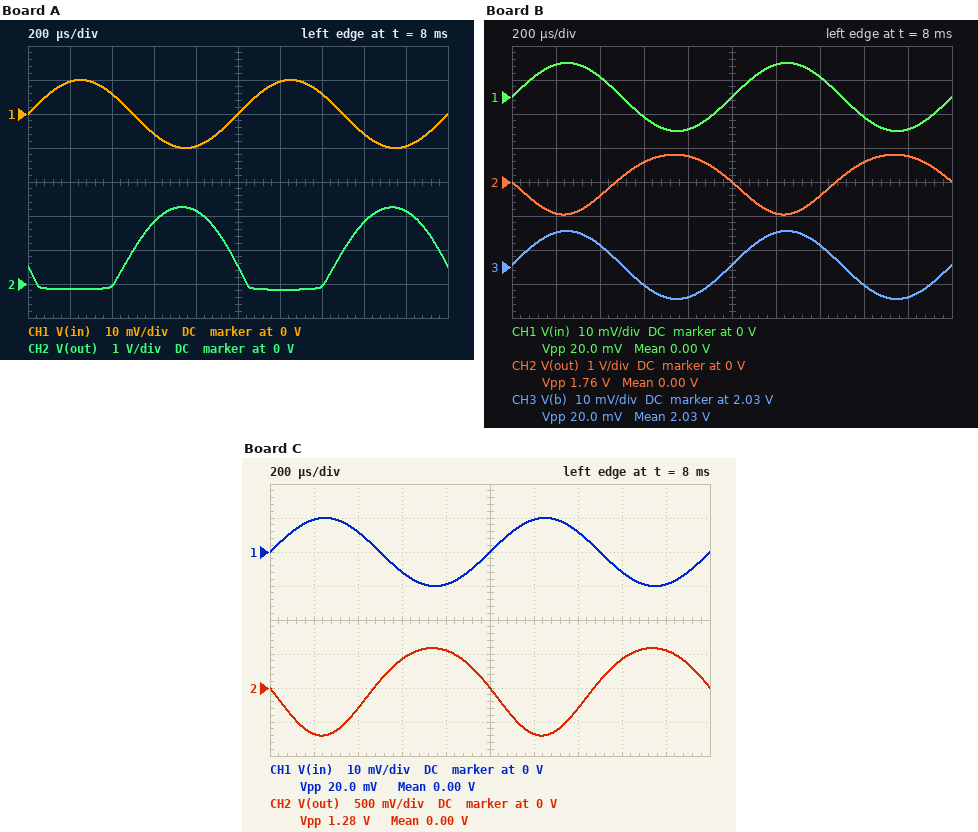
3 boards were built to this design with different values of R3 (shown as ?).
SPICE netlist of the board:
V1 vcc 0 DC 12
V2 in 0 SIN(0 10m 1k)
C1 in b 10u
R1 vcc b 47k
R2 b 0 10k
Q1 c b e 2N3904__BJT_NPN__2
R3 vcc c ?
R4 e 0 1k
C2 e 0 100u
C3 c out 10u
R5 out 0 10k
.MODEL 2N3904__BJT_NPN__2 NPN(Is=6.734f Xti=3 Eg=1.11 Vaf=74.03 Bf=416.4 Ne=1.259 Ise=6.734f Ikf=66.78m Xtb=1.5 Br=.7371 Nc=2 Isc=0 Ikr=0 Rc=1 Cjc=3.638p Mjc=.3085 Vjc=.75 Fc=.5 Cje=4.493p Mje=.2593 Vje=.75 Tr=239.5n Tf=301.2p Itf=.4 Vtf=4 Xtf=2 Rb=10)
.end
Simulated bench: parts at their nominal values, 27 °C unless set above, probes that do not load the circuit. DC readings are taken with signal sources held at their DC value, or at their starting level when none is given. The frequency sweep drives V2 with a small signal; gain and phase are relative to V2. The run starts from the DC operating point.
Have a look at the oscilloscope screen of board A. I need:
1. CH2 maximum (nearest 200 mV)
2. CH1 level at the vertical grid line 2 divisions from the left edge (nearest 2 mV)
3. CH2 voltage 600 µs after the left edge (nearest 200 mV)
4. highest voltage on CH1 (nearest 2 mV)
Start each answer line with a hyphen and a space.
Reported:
- 2.2 V
- 6 mV
- 1.8 V
- 10 mV
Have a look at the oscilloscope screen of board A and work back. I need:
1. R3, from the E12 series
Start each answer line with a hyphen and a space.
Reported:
- 8.2 kΩ
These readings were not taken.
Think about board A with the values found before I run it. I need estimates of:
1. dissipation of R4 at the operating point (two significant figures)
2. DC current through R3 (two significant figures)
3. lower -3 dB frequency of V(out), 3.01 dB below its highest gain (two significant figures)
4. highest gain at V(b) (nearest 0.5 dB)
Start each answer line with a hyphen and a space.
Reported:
- 1.7 mW
- 1.3 mA
- 300 Hz
- 0 dB
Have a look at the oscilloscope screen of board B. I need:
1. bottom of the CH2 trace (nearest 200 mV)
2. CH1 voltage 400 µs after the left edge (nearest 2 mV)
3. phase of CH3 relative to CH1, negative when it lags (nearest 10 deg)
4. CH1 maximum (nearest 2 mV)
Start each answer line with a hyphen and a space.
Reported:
- -1.0 V
- 6 mV
- 0 deg
- 10 mV
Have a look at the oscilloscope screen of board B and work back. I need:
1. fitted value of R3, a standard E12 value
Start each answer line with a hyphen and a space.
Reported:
- 2.2 kΩ
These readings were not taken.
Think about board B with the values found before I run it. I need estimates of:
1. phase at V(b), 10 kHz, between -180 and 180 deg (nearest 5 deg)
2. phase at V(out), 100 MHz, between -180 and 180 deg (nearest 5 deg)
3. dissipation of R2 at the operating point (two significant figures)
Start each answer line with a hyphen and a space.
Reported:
- 0 deg
- 100 deg
- 410 µW
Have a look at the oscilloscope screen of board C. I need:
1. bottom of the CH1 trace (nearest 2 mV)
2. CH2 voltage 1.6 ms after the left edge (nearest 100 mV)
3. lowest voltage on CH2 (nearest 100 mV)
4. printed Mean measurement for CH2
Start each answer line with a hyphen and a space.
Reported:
- -10 mV
- 400 mV
- -700 mV
- 0.00 V
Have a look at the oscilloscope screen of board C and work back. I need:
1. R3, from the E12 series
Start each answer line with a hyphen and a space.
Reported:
- 1.5 kΩ
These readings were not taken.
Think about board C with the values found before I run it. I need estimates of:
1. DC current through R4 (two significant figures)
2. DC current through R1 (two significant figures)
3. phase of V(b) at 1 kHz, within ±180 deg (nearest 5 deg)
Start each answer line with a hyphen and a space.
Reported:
- 1.4 mA
- 210 µA
- 0 deg
